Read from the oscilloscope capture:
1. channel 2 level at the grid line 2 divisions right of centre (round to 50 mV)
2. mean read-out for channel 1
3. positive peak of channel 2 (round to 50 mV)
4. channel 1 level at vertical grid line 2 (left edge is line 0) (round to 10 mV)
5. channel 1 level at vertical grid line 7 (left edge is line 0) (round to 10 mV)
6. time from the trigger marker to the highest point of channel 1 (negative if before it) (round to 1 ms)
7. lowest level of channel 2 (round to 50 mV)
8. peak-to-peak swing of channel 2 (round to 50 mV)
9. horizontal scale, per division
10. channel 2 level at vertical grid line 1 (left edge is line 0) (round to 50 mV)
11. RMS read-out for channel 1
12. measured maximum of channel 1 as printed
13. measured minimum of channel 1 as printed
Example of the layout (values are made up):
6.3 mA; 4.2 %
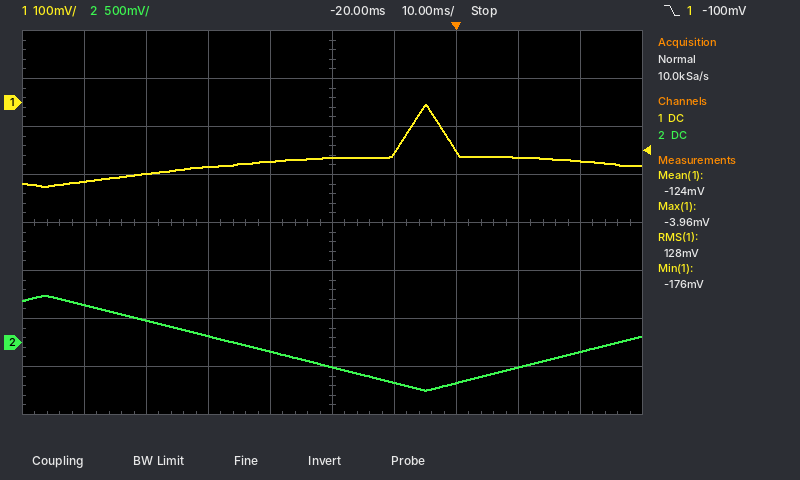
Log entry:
-400 mV; -124 mV; 500 mV; -150 mV; -100 mV; -5 ms; -500 mV; 1.00 V; 10 ms; 400 mV; 128 mV; -3.96 mV; -176 mV
